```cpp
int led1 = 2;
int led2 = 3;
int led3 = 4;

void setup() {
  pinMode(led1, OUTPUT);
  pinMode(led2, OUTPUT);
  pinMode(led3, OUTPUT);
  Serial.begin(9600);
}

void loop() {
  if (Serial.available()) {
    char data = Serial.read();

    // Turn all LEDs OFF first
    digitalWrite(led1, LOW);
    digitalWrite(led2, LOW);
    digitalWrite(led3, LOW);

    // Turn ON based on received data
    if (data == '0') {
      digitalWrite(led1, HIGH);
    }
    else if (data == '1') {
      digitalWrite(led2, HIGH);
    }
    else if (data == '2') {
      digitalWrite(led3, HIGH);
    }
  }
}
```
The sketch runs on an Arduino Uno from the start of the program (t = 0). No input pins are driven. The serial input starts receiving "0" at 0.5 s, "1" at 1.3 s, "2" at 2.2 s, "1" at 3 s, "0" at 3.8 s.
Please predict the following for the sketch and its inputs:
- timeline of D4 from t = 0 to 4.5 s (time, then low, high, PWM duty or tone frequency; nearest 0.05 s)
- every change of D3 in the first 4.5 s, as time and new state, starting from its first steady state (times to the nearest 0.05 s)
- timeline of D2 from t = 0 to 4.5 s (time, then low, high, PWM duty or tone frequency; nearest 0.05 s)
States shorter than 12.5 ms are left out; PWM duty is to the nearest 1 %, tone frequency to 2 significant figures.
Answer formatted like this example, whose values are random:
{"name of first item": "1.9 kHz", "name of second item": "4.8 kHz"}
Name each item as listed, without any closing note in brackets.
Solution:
{"timeline of D4 from t = 0 to 4.5 s": "0 s low; 2.2 s high; 3 s low", "every change of D3 in the first 4.5 s, as time and new state, starting from its first steady state": "0 s low; 1.3 s high; 2.2 s low; 3 s high; 3.8 s low", "timeline of D2 from t = 0 to 4.5 s": "0 s low; 0.5 s high; 1.3 s low; 3.8 s high"}
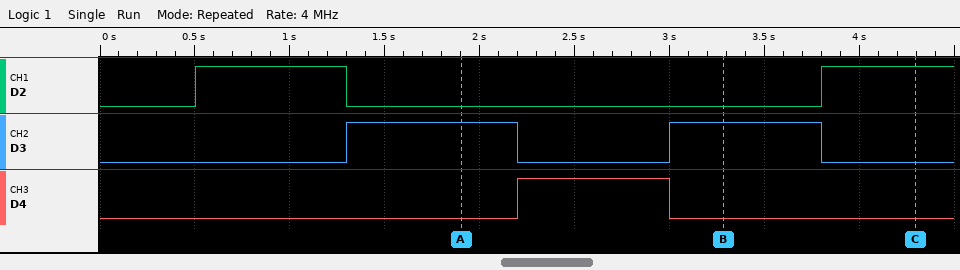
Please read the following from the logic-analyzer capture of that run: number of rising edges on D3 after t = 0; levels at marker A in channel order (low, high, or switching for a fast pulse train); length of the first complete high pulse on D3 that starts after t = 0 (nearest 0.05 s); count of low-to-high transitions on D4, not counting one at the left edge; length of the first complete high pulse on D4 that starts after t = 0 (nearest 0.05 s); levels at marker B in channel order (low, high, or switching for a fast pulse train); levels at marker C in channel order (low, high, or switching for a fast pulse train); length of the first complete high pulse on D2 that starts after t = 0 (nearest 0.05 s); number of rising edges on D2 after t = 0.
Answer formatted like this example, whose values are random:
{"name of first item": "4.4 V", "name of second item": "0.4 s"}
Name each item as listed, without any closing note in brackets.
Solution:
{"number of rising edges on D3 after t = 0": "2", "levels at marker A in channel order": "D2 low, D3 high, D4 low", "length of the first complete high pulse on D3 that starts after t = 0": "0.90 s", "count of low-to-high transitions on D4, not counting one at the left edge": "1", "length of the first complete high pulse on D4 that starts after t = 0": "0.80 s", "levels at marker B in channel order": "D2 low, D3 high, D4 low", "levels at marker C in channel order": "D2 high, D3 low, D4 low", "length of the first complete high pulse on D2 that starts after t = 0": "0.80 s", "number of rising edges on D2 after t = 0": "2"}
